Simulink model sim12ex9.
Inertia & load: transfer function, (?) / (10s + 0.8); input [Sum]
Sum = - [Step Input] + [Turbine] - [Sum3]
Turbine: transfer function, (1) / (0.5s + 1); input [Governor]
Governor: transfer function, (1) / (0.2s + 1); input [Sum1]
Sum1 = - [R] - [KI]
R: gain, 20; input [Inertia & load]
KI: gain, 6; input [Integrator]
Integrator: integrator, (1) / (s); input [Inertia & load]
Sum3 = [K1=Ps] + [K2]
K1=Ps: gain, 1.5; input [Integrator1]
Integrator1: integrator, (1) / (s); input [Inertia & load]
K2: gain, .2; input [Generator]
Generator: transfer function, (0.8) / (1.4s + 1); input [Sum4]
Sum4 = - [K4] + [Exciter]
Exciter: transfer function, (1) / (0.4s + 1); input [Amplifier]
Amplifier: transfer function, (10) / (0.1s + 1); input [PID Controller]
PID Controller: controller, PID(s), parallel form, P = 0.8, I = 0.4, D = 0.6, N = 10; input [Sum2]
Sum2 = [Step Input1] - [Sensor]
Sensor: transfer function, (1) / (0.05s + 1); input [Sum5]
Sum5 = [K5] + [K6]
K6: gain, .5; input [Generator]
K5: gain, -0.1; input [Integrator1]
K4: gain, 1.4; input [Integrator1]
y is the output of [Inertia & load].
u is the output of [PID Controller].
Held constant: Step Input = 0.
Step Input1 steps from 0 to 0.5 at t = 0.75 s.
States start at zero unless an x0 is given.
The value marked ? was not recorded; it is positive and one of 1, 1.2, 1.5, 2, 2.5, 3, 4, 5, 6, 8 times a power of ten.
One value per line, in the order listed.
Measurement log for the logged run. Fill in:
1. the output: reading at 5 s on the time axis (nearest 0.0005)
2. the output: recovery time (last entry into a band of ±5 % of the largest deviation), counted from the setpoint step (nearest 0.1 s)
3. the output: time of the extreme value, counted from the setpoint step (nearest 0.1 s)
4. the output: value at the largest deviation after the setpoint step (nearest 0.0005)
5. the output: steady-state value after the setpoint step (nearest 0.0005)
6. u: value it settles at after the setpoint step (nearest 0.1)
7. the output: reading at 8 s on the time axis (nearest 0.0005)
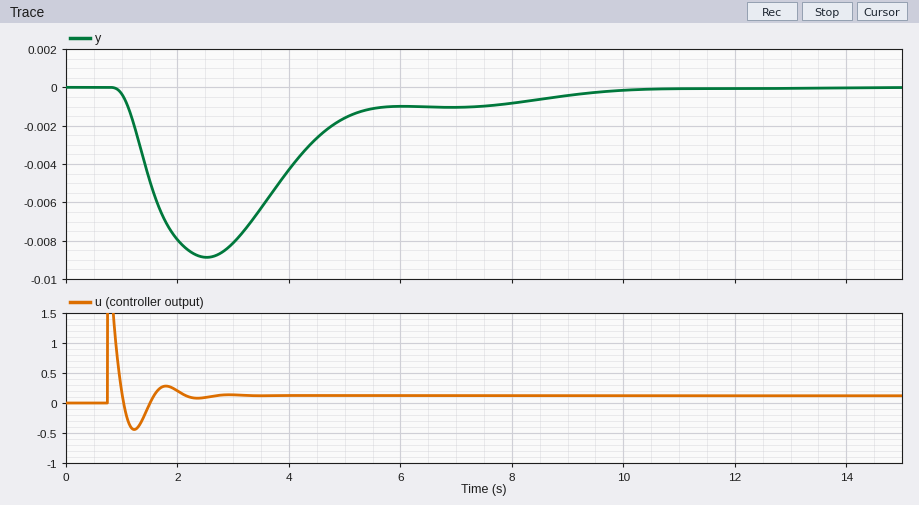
-0.0015
8.2 s
1.8 s
-0.0090
0.0000
0.1
-0.0010
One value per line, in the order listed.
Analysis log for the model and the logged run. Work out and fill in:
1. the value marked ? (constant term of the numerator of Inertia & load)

0.6
